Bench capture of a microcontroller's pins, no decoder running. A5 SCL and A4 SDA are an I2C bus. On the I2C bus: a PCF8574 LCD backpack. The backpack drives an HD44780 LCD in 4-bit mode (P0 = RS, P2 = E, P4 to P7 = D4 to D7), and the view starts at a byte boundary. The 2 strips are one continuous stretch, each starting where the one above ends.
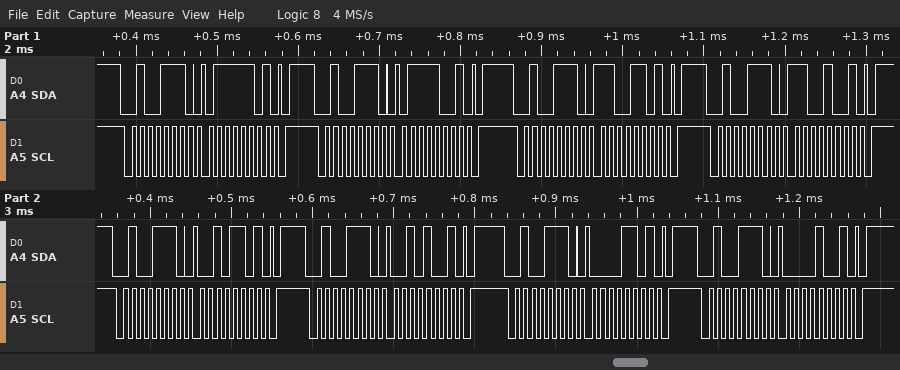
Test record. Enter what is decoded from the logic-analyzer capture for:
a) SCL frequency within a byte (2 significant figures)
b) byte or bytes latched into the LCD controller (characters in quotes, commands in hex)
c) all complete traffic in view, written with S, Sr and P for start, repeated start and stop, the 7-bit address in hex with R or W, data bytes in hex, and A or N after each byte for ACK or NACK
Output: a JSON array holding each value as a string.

["100 kHz", "'|' ' '", "S 27W A 7D A P S 27W A 79 A P S 27W A CD A P S 27W A C9 A P S 27W A 2D A P S 27W A 29 A P S 27W A 0D A P S 27W A 09 A P"]
